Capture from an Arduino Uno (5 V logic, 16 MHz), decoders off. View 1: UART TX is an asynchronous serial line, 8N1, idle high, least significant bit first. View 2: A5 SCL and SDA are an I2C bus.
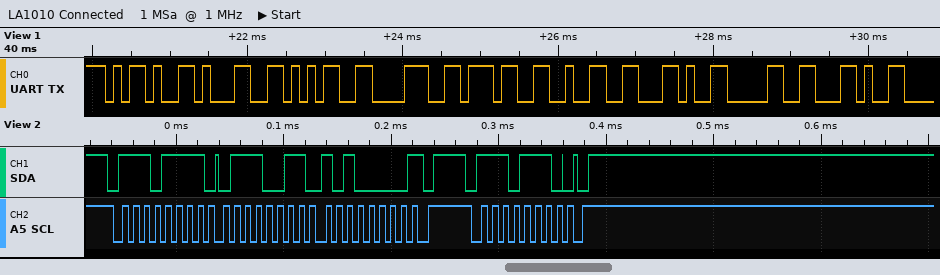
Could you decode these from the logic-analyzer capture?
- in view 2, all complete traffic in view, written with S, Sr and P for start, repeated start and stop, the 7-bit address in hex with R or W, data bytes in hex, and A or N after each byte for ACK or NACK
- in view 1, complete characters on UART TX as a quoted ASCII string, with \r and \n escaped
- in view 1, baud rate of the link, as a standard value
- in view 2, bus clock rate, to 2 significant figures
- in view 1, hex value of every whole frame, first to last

S 77R A 73 A A0 N P S 77W A P
"-15872,0,"
9600 baud
100 kHz
2D 31 35 38 37 32 2C 30 2C
